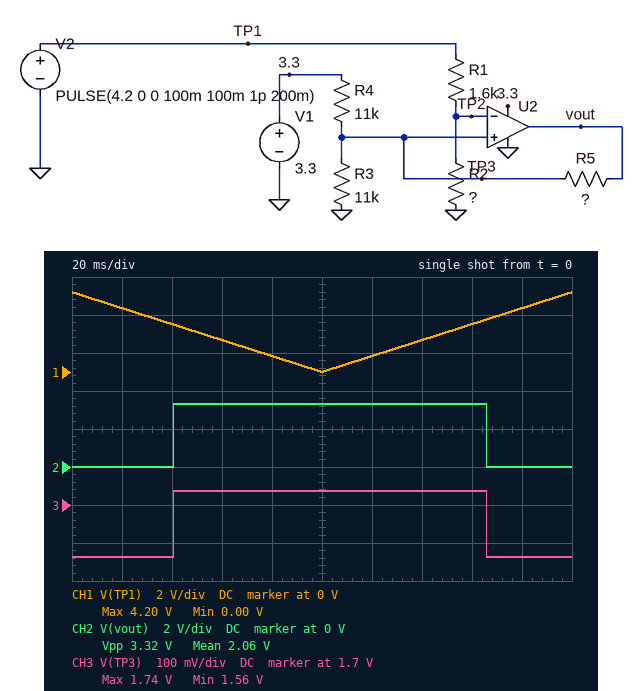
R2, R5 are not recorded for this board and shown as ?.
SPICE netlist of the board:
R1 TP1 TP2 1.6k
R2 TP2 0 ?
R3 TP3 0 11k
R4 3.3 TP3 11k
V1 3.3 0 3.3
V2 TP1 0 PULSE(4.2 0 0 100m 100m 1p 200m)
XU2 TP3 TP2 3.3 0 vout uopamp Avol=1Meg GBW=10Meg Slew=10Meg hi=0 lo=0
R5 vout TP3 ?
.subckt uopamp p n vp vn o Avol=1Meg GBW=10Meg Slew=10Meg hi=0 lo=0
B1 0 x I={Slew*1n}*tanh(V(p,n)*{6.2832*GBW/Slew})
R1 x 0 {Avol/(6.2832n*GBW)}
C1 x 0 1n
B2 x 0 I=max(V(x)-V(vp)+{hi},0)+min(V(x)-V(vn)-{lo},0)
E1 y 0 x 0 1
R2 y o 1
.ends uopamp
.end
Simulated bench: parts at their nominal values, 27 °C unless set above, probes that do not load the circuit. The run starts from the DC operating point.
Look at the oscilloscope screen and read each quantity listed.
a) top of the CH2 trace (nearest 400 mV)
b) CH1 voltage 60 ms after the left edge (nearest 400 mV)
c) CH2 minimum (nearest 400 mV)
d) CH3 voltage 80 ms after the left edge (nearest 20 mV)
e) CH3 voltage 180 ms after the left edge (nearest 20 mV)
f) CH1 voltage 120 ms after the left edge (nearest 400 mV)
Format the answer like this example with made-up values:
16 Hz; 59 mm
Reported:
3.2 V; 1.6 V; 0 V; 1.74 V; 1.56 V; 800 mV
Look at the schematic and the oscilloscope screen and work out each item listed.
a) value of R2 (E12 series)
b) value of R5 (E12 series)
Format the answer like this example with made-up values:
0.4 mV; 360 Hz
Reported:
2.7 kΩ; 100 kΩ
